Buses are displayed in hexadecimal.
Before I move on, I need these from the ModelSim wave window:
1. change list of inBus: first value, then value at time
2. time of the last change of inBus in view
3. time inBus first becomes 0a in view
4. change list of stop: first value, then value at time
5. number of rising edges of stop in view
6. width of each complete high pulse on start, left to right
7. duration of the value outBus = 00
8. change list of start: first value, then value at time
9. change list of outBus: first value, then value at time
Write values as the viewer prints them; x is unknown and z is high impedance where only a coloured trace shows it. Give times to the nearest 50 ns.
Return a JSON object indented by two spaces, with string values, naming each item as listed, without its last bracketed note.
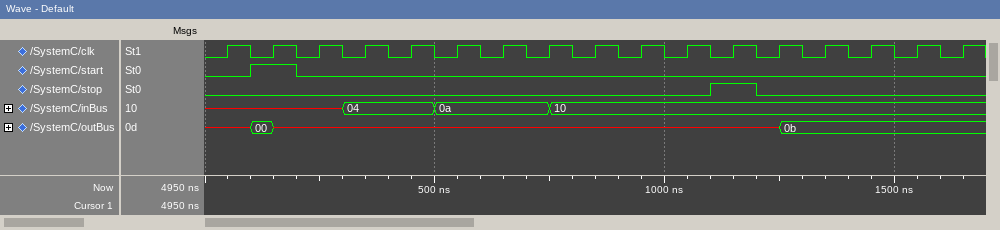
{
  "change list of inBus: first value, then value at time": "x, 04 at 300 ns, 0a at 500 ns, 10 at 750 ns",
  "time of the last change of inBus in view": "750 ns",
  "time inBus first becomes 0a in view": "500 ns",
  "change list of stop: first value, then value at time": "0, 1 at 1100 ns, 0 at 1200 ns",
  "number of rising edges of stop in view": "1",
  "width of each complete high pulse on start, left to right": "100 ns",
  "duration of the value outBus = 00": "50 ns",
  "change list of start: first value, then value at time": "0, 1 at 100 ns, 0 at 200 ns",
  "change list of outBus: first value, then value at time": "x, 00 at 100 ns, x at 150 ns, 0b at 1250 ns"
}
